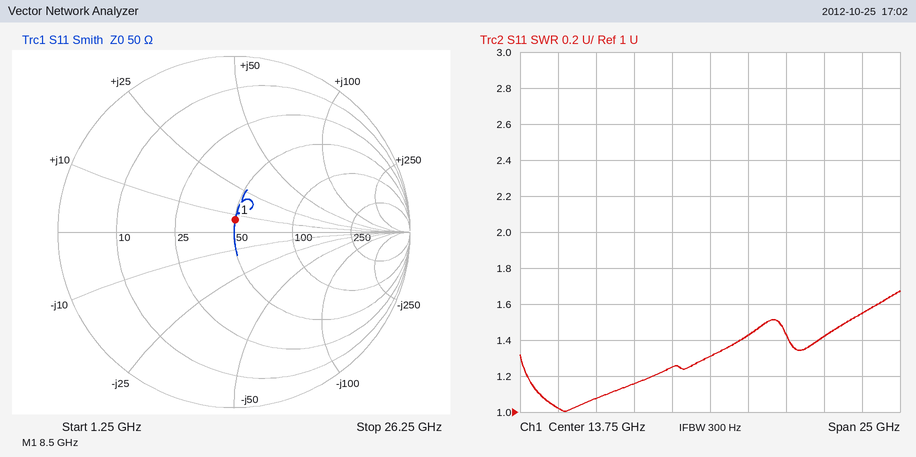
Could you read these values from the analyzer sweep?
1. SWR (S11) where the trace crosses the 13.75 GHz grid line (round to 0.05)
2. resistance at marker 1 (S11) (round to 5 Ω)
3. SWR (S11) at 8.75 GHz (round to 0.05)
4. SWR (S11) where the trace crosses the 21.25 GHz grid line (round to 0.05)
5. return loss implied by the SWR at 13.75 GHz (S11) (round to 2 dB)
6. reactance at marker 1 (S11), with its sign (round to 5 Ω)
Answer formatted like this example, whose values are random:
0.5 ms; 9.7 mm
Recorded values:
1.30; 50 Ω; 1.15; 1.40; 18 dB; +5 Ω
